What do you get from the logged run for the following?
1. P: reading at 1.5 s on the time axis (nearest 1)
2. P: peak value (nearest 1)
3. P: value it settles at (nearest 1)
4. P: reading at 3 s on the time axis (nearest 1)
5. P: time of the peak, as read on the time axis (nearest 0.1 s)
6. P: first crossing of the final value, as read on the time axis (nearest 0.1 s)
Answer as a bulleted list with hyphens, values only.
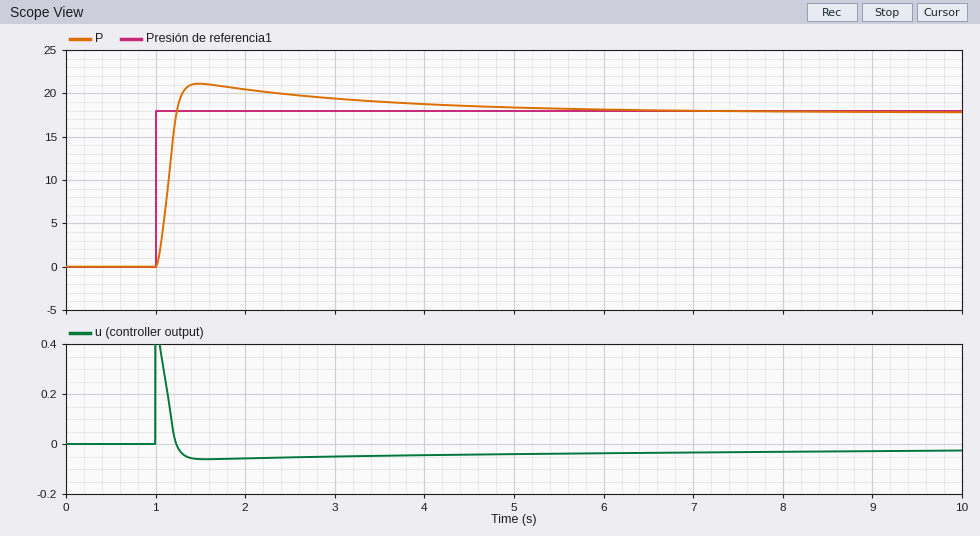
- 21
- 21
- 18
- 19
- 1.5 s
- 1.2 s
